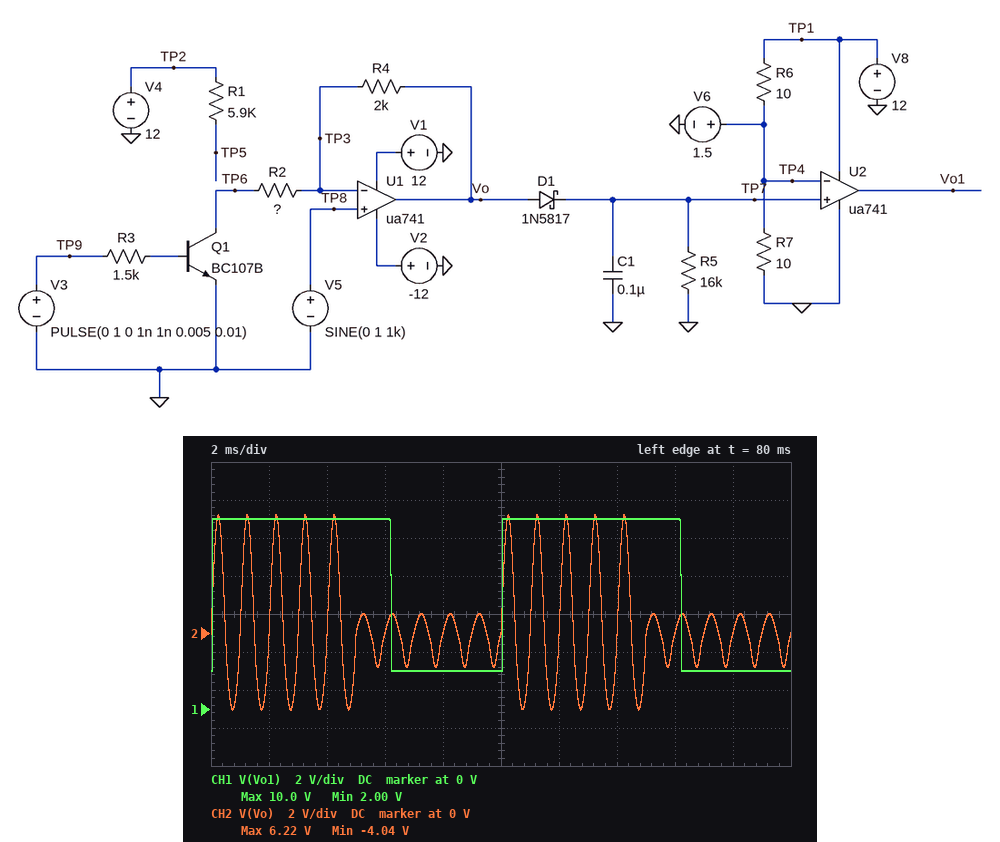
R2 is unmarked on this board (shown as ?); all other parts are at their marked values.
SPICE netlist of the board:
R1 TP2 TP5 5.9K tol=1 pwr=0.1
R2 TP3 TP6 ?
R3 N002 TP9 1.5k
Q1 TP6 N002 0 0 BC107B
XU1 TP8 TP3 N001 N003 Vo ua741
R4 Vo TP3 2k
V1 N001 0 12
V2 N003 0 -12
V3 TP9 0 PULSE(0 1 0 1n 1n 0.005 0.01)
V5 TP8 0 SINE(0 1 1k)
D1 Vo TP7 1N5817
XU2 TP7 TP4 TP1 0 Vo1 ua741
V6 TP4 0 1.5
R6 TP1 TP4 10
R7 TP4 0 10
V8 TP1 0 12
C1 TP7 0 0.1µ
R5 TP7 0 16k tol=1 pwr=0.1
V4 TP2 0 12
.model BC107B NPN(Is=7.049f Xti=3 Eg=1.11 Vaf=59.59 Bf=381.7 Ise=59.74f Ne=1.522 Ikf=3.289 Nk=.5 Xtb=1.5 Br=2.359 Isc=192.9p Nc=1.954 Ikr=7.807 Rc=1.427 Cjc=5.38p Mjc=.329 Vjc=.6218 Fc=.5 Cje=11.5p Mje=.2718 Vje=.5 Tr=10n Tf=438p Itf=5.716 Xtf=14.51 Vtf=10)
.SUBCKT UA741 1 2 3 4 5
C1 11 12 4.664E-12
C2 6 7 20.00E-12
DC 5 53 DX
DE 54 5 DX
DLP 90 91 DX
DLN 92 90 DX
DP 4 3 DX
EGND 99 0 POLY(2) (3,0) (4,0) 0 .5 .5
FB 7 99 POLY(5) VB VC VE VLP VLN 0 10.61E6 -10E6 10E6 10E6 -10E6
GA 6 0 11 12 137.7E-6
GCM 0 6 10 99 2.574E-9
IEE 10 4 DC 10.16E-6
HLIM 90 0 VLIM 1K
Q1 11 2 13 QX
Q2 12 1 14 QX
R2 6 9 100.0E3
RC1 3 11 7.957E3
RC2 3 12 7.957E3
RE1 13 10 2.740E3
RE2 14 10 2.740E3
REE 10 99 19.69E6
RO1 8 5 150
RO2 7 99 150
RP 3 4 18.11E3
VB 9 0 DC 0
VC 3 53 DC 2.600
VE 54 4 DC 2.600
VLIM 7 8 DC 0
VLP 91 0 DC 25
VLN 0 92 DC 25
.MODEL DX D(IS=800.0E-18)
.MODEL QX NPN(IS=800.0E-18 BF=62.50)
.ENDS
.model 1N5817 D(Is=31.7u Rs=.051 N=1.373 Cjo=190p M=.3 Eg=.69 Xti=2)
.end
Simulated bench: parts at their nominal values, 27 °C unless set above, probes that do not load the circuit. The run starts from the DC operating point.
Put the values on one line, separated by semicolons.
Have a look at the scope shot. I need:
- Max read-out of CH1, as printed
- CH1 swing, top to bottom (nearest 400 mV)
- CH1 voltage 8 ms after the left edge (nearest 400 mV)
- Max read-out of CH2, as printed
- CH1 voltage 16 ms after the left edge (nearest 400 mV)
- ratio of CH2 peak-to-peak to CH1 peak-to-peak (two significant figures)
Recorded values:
10.0 V; 8.0 V; 2.0 V; 6.22 V; 10.0 V; 1.3
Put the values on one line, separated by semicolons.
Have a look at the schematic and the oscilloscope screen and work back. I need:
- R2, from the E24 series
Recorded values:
360 Ω
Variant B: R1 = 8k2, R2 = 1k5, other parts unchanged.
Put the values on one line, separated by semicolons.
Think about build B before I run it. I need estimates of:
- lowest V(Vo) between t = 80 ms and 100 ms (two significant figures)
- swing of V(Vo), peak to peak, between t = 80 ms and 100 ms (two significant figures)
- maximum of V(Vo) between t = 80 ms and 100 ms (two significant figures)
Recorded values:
-2.3 V; 4.6 V; 2.3 V
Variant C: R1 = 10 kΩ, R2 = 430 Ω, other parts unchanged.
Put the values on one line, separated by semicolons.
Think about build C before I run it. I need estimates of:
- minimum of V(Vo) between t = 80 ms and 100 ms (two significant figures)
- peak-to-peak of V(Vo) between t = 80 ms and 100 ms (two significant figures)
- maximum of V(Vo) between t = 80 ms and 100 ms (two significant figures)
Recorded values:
-3.8 V; 9.2 V; 5.4 V
